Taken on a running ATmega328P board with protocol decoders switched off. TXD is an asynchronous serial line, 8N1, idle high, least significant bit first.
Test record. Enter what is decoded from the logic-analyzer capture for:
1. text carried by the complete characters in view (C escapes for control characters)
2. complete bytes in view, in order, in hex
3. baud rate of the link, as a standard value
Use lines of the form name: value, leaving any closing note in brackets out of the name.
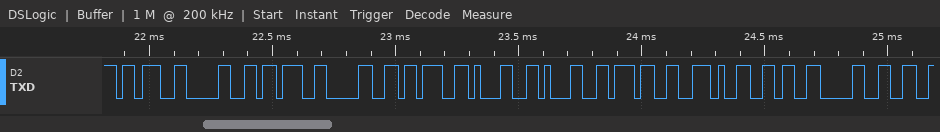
text carried by the complete characters in view: ";0;0;117.60"
complete bytes in view, in order, in hex: 0x3B 0x30 0x3B 0x30 0x3B 0x31 0x31 0x37 0x2E 0x36 0x30
baud rate of the link, as a standard value: 38400 baud
